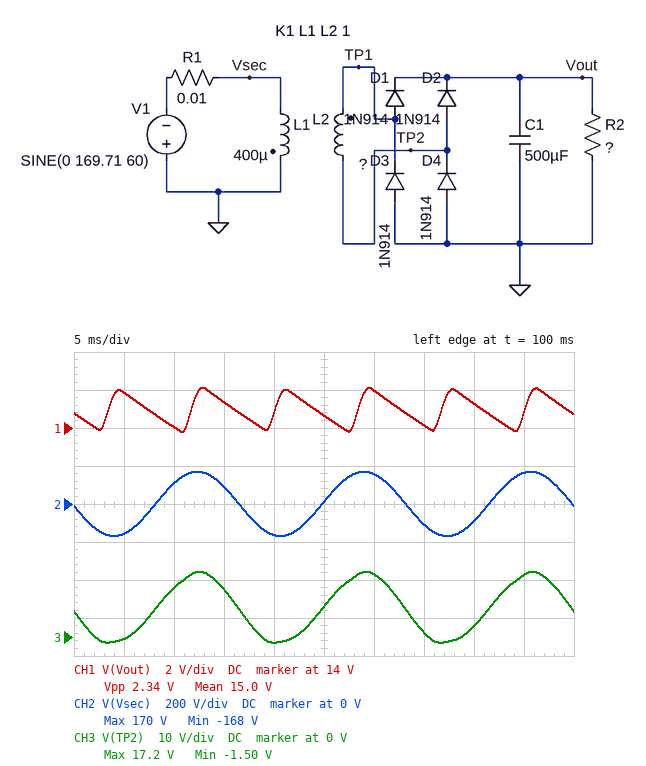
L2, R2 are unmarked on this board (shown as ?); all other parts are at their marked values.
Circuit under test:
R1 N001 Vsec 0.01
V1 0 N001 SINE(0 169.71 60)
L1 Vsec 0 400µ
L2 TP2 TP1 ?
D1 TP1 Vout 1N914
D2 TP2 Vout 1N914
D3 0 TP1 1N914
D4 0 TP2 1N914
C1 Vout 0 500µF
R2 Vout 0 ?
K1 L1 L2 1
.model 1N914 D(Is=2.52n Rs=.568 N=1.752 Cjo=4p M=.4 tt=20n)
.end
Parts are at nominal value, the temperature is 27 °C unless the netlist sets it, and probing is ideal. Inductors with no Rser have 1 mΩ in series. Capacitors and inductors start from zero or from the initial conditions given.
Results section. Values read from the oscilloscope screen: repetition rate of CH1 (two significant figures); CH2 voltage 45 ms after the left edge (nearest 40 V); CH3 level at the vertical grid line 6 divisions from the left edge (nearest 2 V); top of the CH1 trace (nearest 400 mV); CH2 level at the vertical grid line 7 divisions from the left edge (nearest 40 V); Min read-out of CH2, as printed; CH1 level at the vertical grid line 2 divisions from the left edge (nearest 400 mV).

120 Hz
160 V
16 V
16.0 V
-120 V
-168 V
14.0 V
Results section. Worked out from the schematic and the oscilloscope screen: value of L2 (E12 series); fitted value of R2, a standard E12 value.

4.7 µH
82 Ω
